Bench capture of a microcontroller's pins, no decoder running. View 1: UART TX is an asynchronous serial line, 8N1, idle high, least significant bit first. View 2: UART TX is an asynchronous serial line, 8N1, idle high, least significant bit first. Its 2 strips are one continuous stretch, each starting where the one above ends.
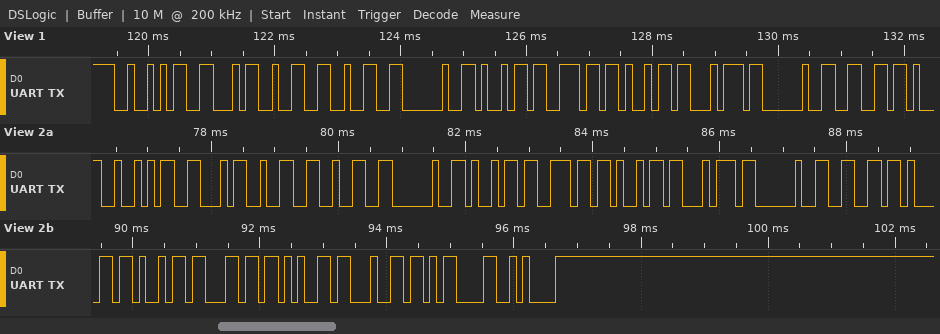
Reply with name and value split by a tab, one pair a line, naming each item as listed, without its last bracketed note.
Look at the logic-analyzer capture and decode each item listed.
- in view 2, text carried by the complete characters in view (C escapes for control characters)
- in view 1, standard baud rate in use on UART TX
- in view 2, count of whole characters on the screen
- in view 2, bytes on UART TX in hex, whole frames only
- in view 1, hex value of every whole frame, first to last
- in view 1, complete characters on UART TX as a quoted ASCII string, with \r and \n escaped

in view 2, text carried by the complete characters in view	"RF22 init failed\r\n"
in view 1, standard baud rate in use on UART TX	9600 baud
in view 2, count of whole characters on the screen	18
in view 2, bytes on UART TX in hex, whole frames only	52 46 32 32 20 69 6E 69 74 20 66 61 69 6C 65 64 0D 0A
in view 1, hex value of every whole frame, first to last	52 46 32 32 20 69 6E 69 74 20 66
in view 1, complete characters on UART TX as a quoted ASCII string, with \r and \n escaped	"RF22 init f"
